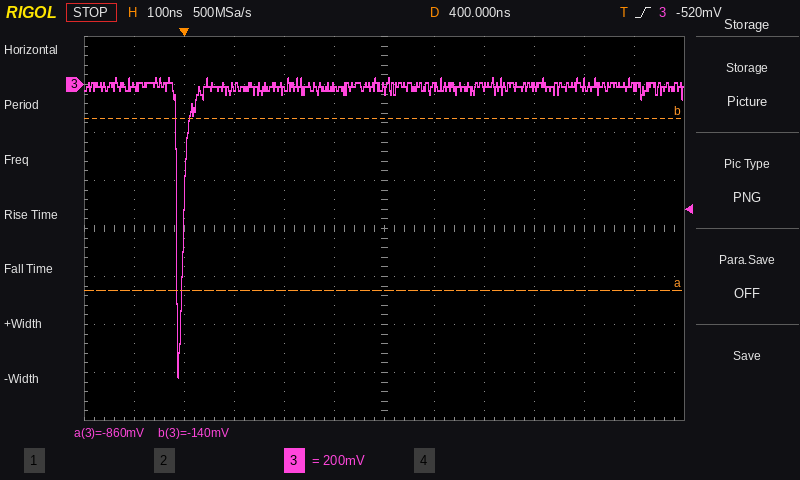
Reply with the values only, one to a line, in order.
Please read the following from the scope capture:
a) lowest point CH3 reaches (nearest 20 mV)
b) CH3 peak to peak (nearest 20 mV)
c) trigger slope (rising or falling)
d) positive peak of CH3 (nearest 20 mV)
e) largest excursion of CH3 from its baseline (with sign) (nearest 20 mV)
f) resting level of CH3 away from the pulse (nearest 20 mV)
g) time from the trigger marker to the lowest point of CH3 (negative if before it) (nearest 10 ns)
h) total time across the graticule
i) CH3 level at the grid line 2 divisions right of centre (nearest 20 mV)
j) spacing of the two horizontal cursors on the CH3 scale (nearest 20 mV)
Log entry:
-1.22 V
1.24 V
rising
20 mV
-1.22 V
0 mV
-10 ns
1.2 µs
0 mV
720 mV
